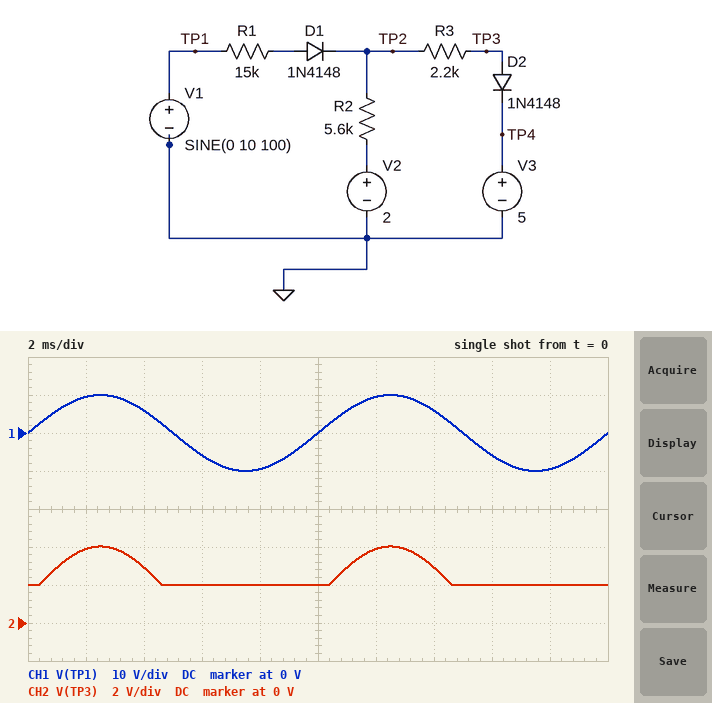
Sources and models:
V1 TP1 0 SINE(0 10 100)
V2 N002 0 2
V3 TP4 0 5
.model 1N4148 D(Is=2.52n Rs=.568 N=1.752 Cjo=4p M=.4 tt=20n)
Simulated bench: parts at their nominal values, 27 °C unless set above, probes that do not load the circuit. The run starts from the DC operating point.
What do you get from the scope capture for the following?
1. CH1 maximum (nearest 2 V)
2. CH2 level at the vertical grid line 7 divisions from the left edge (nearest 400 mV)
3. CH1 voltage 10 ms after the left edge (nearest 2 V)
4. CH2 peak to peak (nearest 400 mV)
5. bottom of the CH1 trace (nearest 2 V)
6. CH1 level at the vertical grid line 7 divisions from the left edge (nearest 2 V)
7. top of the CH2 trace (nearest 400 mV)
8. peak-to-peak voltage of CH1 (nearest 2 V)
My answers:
10 V
2.8 V
0 V
2.0 V
-10 V
6 V
4.0 V
20 V
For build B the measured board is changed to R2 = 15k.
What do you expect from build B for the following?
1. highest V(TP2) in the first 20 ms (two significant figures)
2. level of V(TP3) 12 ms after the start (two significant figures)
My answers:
5.5 V
5.4 V
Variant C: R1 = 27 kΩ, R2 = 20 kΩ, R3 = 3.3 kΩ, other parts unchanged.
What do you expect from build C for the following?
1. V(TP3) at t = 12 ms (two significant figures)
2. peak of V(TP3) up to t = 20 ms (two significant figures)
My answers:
5.0 V
5.2 V
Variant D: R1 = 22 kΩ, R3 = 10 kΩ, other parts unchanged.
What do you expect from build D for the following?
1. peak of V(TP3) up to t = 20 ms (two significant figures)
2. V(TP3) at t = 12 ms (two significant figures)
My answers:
3.5 V
3.4 V
